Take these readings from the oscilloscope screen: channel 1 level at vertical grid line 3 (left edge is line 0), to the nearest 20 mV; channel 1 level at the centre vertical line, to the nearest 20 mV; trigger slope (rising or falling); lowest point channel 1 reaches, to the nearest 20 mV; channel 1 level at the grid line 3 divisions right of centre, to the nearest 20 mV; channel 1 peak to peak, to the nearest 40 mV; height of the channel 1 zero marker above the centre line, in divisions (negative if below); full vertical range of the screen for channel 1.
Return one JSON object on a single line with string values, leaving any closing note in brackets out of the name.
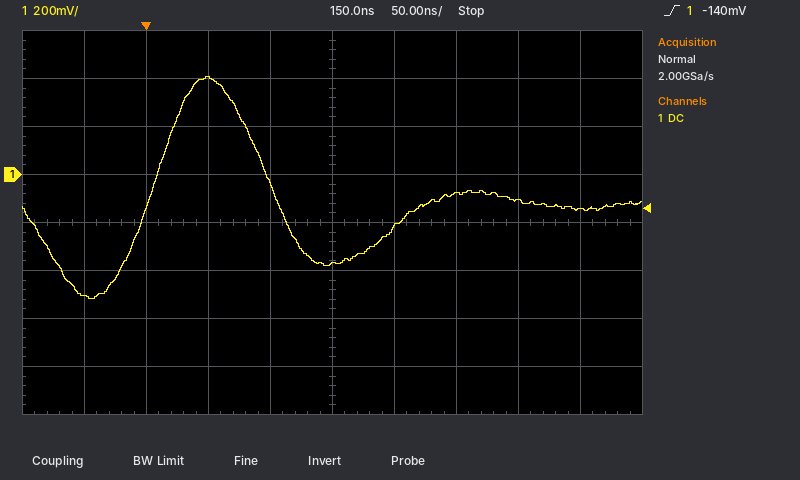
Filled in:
{"channel 1 level at vertical grid line 3 (left edge is line 0), to the nearest 20 mV": "400 mV", "channel 1 level at the centre vertical line, to the nearest 20 mV": "-380 mV", "trigger slope": "rising", "lowest point channel 1 reaches, to the nearest 20 mV": "-520 mV", "channel 1 level at the grid line 3 divisions right of centre, to the nearest 20 mV": "-100 mV", "channel 1 peak to peak, to the nearest 40 mV": "920 mV", "height of the channel 1 zero marker above the centre line, in divisions": "+1.0 div", "full vertical range of the screen for channel 1": "1.6 V"}
